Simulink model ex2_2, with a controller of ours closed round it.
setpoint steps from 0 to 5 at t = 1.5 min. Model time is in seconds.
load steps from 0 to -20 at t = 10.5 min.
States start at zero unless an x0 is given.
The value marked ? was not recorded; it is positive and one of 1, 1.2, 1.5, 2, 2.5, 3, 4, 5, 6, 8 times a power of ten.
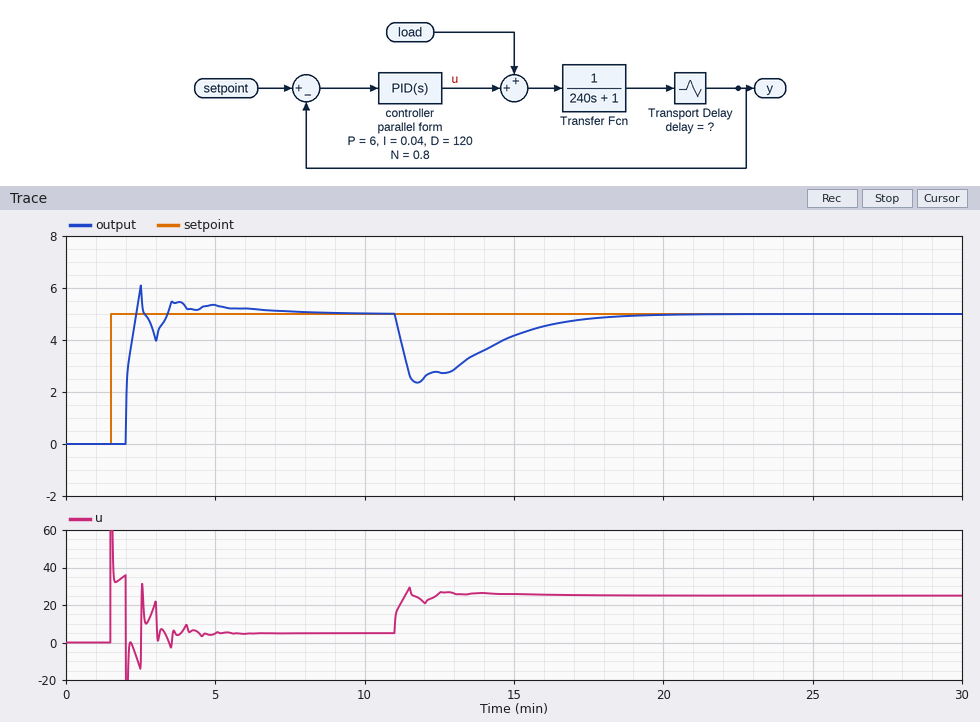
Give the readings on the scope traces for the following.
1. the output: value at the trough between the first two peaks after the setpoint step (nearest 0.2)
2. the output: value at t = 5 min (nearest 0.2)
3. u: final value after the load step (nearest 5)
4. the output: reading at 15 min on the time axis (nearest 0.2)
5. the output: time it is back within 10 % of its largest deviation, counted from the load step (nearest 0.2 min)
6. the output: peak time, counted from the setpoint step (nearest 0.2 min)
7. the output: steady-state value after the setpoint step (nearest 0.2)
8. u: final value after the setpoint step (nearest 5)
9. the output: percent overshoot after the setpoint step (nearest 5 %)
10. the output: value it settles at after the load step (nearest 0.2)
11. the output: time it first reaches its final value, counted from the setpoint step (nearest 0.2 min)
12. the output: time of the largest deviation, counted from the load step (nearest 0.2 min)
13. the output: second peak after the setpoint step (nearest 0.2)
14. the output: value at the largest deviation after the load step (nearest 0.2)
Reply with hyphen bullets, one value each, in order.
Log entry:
- 4.0
- 5.4
- 25
- 4.2
- 6.4 min
- 1.0 min
- 5.0
- 5
- 20 %
- 5.0
- 0.8 min
- 1.2 min
- 5.4
- 2.4
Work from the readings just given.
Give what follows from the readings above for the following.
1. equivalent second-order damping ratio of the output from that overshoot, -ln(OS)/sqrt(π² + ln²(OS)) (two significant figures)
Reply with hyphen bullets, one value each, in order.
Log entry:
- 0.46
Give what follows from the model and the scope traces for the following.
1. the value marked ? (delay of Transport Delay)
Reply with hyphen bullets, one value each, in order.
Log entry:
- 30
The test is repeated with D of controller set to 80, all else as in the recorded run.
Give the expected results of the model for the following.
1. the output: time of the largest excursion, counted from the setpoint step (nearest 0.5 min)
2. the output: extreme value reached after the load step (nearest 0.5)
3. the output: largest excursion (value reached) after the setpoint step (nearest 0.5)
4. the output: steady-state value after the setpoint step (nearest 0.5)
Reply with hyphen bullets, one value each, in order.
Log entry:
- 2.5 min
- 2.0
- 5.5
- 5.0
